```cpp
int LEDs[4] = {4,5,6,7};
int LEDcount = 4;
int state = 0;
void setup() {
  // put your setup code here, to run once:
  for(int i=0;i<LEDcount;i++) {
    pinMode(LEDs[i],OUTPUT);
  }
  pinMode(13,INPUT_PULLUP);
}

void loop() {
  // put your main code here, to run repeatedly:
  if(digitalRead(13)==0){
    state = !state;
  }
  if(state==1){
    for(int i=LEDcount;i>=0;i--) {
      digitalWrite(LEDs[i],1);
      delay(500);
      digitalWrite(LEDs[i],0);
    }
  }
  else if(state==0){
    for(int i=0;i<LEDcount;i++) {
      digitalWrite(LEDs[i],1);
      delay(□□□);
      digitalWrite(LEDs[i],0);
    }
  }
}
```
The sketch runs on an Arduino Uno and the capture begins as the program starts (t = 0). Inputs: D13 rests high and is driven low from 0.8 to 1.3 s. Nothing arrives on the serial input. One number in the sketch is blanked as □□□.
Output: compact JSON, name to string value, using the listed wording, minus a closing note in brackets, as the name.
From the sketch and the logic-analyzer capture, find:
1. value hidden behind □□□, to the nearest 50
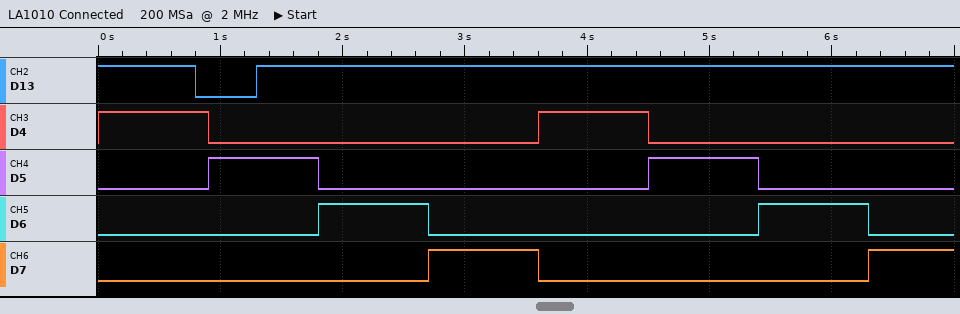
{"value hidden behind □□□, to the nearest 50": "900"}
